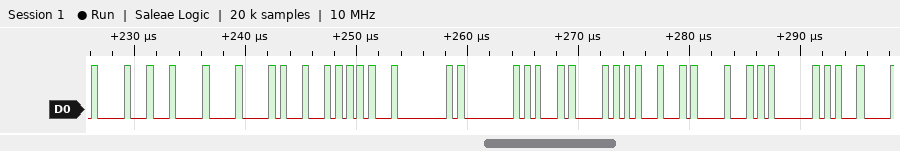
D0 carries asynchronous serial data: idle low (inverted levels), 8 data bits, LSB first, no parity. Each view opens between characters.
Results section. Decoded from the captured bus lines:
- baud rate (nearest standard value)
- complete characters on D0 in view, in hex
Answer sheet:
2000000 baud
DF, F7, DF, DD, 55, FF, FD, 75, 5F, DD, 7D, F5, 75
